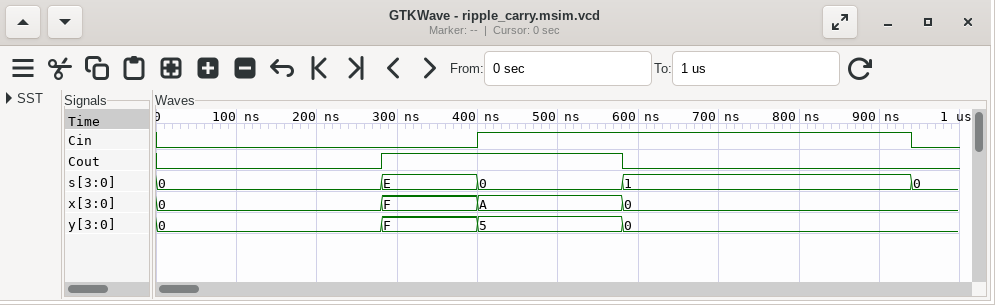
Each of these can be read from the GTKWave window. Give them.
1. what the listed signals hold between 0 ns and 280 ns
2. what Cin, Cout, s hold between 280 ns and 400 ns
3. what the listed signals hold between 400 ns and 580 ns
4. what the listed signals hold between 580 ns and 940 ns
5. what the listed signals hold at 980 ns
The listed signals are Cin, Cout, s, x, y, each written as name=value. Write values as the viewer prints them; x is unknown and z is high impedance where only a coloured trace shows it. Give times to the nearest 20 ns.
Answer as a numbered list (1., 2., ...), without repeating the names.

1. Cin=0, Cout=0, s=0, x=0, y=0
2. Cin=0, Cout=1, s=E
3. Cin=1, Cout=1, s=0, x=A, y=5
4. Cin=1, Cout=0, s=1, x=0, y=0
5. Cin=0, Cout=0, s=0, x=0, y=0
